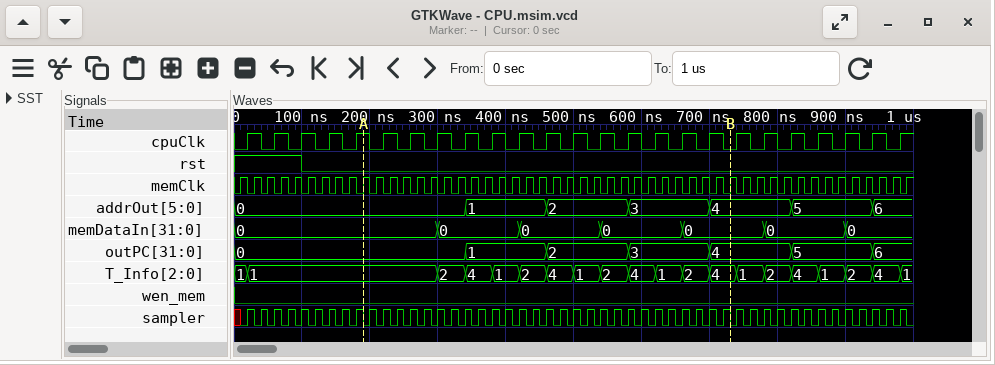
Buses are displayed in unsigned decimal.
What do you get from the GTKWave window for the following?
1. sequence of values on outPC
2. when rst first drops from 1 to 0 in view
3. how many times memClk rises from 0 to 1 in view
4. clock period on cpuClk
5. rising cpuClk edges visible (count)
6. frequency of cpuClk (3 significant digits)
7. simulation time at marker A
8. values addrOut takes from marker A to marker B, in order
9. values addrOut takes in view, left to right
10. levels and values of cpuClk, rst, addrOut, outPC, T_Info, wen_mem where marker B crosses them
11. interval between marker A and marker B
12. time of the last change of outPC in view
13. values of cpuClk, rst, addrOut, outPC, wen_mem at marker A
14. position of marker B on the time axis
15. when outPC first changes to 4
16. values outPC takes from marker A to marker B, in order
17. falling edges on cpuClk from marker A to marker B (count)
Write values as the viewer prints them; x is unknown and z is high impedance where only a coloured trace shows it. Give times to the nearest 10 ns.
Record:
0, 1, 2, 3, 4, 5, 6
100 ns
50
40 ns
25
25.0 MHz
190 ns
0, 1, 2, 3, 4
0, 1, 2, 3, 4, 5, 6
cpuClk=0, rst=0, addrOut=4, outPC=4, T_Info=4, wen_mem=0
540 ns
940 ns
cpuClk=1, rst=0, addrOut=0, outPC=0, wen_mem=0
730 ns
700 ns
0, 1, 2, 3, 4
14
